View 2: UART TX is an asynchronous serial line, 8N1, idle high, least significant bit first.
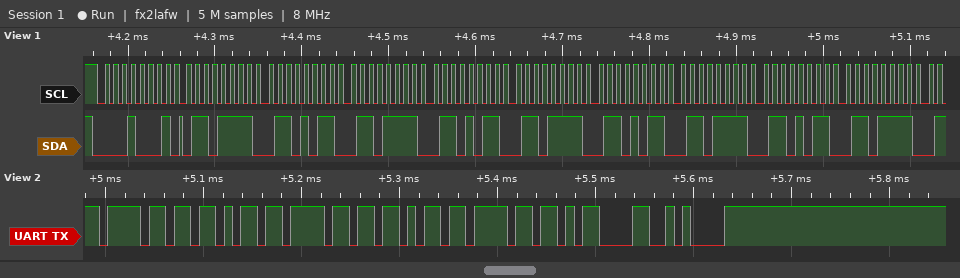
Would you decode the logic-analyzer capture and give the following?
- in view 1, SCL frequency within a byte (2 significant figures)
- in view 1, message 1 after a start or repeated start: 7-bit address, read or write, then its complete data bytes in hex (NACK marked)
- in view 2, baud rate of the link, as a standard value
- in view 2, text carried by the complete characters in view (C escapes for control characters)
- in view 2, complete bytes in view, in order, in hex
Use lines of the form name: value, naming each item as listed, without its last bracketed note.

in view 1, SCL frequency within a byte: 100 kHz
in view 1, message 1 after a start or repeated start: 7-bit address, read or write, then its complete data bytes in hex: 0x08 read: 6F 6B 6F 6B 6F 6B 6F 6B 6F
in view 2, baud rate of the link, as a standard value: 115200 baud
in view 2, text carried by the complete characters in view: "okoko\r\n"
in view 2, complete bytes in view, in order, in hex: 6F 6B 6F 6B 6F 0D 0A
